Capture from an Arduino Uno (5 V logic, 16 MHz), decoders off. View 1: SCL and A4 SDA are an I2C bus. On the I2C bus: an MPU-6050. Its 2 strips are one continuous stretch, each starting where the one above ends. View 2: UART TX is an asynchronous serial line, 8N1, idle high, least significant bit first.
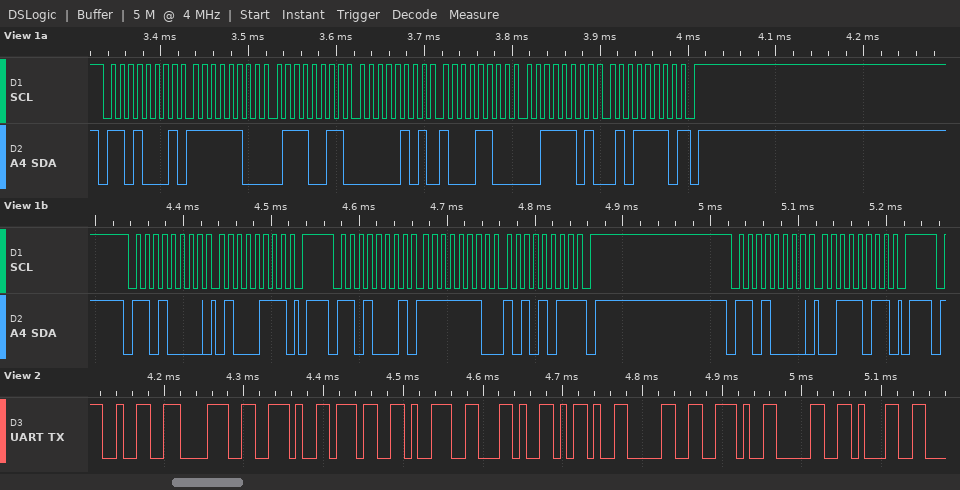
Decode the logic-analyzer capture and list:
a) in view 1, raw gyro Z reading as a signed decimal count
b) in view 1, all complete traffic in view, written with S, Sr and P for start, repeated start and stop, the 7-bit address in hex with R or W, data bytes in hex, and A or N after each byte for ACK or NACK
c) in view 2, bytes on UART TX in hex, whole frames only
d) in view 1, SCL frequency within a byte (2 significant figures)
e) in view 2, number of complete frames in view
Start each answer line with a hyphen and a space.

- -341
- S 68R A FC A 73 A 05 A 8C A 3D A 5E N P S 68W A 47 A P S 68R A FE A AB N P S 68W A 3B A P
- 0x32 0x38 0x2E 0x37 0x39 0x2C 0x2D 0x30 0x2E 0x30 0x31
- 100 kHz
- 11
